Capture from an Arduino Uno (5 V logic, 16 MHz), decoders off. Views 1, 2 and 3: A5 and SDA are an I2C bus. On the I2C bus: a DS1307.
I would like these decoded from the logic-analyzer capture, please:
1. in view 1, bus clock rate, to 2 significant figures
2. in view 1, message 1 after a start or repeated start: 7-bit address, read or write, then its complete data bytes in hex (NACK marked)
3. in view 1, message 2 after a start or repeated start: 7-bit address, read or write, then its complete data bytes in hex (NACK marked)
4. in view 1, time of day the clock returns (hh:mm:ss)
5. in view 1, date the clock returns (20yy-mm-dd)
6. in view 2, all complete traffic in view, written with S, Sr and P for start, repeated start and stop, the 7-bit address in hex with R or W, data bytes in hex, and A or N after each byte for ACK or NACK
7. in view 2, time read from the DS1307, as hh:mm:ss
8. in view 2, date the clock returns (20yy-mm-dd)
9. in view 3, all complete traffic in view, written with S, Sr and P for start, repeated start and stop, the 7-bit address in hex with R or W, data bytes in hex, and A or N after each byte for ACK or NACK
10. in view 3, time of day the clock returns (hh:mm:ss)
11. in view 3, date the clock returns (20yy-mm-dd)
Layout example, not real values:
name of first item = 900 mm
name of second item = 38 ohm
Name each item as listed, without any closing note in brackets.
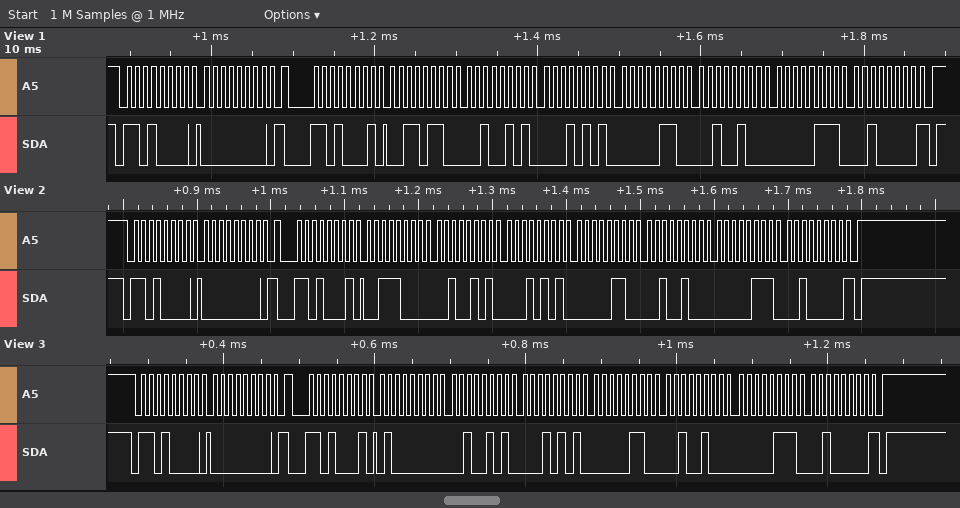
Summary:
in view 1, bus clock rate, to 2 significant figures = 100 kHz
in view 1, message 1 after a start or repeated start: 7-bit address, read or write, then its complete data bytes in hex = 0x68 write: 00
in view 1, message 2 after a start or repeated start: 7-bit address, read or write, then its complete data bytes in hex = 0x68 read: 36 25 15 06 24 07 20 NACK
in view 1, time of day the clock returns = 15:25:36
in view 1, date the clock returns = 2020-07-24
in view 2, all complete traffic in view, written with S, Sr and P for start, repeated start and stop, the 7-bit address in hex with R or W, data bytes in hex, and A or N after each byte for ACK or NACK = S 68W A 00 A Sr 68R A 38 A 25 A 15 A 06 A 24 A 07 A 20 N P
in view 2, time read from the DS1307, as hh:mm:ss = 15:25:38
in view 2, date the clock returns = 2020-07-24
in view 3, all complete traffic in view, written with S, Sr and P for start, repeated start and stop, the 7-bit address in hex with R or W, data bytes in hex, and A or N after each byte for ACK or NACK = S 68W A 00 A Sr 68R A 40 A 25 A 15 A 06 A 24 A 07 A 20 N P
in view 3, time of day the clock returns = 15:25:40
in view 3, date the clock returns = 2020-07-24
